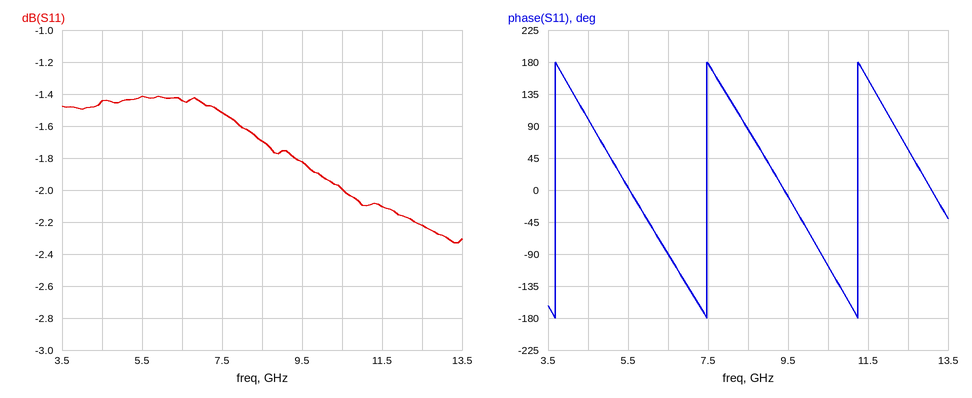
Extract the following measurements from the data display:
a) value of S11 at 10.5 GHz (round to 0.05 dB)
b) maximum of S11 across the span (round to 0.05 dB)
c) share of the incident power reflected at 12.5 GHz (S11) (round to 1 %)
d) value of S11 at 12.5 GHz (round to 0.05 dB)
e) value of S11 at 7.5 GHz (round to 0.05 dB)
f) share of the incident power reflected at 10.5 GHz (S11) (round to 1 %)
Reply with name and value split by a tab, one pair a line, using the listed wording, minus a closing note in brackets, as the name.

value of S11 at 10.5 GHz	-2.00 dB
maximum of S11 across the span	-1.40 dB
share of the incident power reflected at 12.5 GHz (S11)	60 %
value of S11 at 12.5 GHz	-2.20 dB
value of S11 at 7.5 GHz	-1.50 dB
share of the incident power reflected at 10.5 GHz (S11)	63 %
